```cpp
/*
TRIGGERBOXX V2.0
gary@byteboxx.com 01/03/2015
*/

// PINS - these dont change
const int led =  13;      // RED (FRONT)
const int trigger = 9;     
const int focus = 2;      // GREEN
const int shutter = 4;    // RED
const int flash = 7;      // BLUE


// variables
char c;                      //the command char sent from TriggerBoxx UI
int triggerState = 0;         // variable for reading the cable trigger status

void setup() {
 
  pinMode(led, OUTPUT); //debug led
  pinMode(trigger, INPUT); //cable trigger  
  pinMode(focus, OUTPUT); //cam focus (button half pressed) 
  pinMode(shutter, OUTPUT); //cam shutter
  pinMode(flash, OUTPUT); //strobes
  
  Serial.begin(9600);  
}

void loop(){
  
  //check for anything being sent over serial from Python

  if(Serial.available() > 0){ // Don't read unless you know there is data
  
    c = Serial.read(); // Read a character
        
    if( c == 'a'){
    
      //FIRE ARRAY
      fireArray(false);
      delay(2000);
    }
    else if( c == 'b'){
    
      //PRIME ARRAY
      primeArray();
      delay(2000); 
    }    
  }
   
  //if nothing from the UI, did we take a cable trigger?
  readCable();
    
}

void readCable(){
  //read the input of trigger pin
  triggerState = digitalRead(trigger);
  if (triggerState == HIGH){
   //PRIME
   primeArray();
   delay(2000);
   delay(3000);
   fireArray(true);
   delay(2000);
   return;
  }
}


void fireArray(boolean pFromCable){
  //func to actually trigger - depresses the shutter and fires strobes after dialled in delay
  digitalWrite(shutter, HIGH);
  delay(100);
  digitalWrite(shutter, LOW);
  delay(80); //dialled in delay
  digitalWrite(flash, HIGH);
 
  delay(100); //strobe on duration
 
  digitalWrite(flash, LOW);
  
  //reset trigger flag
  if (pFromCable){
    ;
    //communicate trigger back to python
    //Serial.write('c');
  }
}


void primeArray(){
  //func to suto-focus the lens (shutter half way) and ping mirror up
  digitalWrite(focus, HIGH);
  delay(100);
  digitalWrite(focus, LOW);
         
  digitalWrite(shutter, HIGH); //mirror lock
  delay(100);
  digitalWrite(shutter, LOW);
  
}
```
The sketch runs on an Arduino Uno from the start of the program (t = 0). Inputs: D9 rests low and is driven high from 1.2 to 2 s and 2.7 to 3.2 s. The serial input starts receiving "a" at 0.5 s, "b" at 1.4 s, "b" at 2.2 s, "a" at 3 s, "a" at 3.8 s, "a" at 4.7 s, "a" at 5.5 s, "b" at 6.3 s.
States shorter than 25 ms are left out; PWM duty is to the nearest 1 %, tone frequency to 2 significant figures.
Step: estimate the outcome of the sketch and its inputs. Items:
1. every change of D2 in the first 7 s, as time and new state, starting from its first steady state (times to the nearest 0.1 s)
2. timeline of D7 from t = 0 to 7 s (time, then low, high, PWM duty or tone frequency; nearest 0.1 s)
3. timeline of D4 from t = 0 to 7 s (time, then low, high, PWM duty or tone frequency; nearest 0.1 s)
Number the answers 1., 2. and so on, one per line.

1. 0 s low; 2.8 s high; 2.9 s low
2. 0 s low; 0.7 s high; 0.8 s low
3. 0 s low; 0.5 s high; 0.6 s low; 2.9 s high; 3 s low
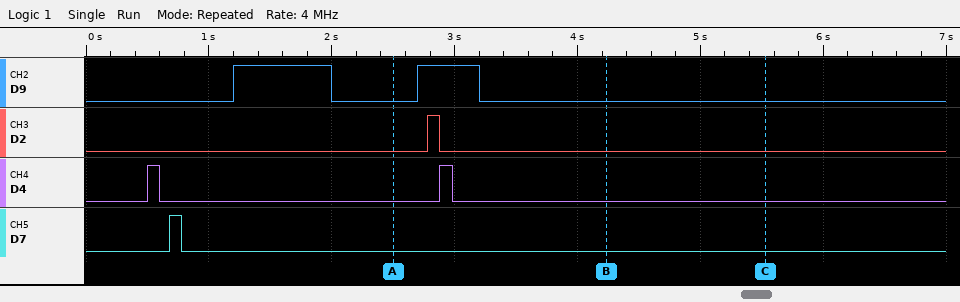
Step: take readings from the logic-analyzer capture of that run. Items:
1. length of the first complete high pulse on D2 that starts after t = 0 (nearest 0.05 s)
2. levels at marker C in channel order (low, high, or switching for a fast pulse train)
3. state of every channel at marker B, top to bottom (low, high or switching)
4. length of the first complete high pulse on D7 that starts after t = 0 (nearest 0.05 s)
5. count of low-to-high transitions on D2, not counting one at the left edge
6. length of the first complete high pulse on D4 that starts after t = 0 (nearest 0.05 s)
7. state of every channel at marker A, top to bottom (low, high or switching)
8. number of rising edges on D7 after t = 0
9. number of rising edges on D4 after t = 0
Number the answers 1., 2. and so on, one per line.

1. 0.10 s
2. D9 low, D2 low, D4 low, D7 low
3. D9 low, D2 low, D4 low, D7 low
4. 0.10 s
5. 1
6. 0.10 s
7. D9 low, D2 low, D4 low, D7 low
8. 1
9. 2
